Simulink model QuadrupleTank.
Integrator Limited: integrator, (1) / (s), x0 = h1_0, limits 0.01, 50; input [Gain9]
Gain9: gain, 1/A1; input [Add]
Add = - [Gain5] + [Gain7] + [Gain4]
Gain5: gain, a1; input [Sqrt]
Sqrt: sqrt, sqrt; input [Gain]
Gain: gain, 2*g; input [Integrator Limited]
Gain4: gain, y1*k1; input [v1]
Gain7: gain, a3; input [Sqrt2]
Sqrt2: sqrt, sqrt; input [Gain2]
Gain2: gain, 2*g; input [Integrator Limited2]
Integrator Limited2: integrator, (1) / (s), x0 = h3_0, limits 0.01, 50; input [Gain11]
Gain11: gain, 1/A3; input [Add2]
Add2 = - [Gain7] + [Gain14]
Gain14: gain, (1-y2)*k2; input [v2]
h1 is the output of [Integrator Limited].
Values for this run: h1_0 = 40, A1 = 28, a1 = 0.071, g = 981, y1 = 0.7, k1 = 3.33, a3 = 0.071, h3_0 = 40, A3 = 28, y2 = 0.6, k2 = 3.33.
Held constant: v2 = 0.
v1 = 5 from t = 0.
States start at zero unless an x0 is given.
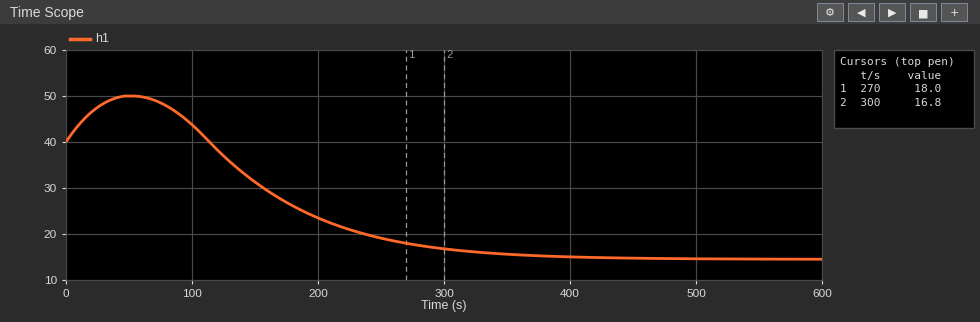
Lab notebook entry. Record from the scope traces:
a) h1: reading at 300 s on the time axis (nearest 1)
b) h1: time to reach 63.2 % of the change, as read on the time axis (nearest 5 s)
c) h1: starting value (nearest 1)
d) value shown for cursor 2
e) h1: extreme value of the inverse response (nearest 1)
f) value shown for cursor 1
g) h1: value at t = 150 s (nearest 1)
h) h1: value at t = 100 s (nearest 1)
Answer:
17
195 s
40
16.8
50
18.0
31
44
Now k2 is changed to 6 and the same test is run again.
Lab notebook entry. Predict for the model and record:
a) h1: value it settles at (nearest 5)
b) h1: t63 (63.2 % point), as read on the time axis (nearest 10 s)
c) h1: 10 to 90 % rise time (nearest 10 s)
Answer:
15
200 s
170 s
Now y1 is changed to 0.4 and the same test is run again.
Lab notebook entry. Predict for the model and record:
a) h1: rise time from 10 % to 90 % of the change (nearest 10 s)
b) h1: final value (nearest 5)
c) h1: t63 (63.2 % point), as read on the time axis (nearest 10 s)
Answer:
130 s
5
150 s
